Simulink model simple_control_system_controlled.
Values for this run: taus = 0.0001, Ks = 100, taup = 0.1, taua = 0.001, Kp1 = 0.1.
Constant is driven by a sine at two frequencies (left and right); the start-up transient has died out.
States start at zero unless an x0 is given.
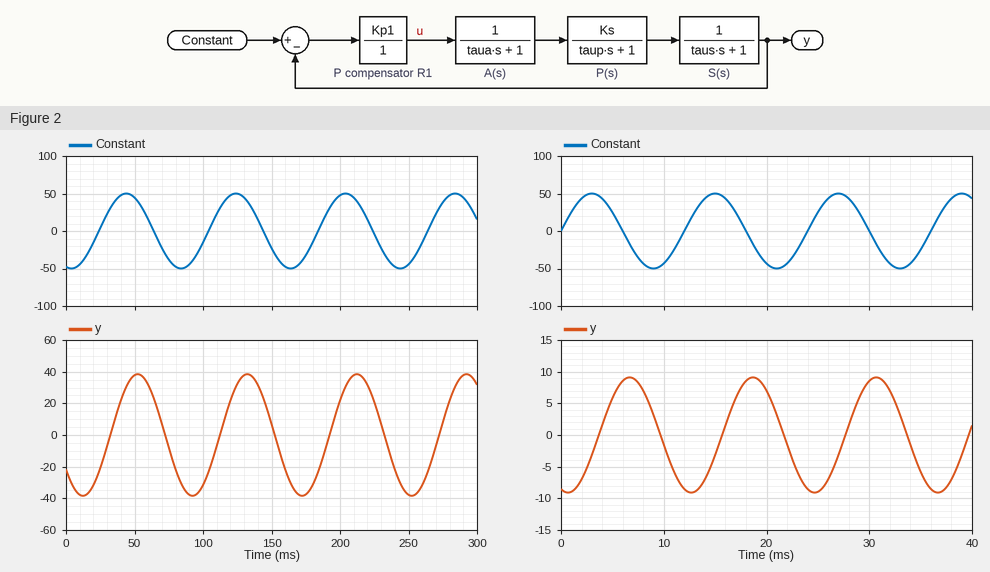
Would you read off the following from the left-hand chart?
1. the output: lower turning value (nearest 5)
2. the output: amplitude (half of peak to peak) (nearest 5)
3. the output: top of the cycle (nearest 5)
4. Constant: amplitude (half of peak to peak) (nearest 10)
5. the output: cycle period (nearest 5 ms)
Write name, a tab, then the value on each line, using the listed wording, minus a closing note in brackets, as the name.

the output: lower turning value	-40
the output: amplitude (half of peak to peak)	40
the output: top of the cycle	40
Constant: amplitude (half of peak to peak)	50
the output: cycle period	80 ms
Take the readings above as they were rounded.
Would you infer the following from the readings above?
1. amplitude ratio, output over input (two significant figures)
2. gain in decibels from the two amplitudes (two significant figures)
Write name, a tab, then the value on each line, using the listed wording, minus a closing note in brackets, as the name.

amplitude ratio, output over input	0.80
gain in decibels from the two amplitudes	-1.9 dB
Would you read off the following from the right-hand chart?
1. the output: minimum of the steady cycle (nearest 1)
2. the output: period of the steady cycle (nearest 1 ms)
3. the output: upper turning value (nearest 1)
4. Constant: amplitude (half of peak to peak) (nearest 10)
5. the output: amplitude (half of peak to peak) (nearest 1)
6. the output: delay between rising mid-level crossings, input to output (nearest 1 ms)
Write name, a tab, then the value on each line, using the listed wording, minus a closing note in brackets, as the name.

the output: minimum of the steady cycle	-9
the output: period of the steady cycle	12 ms
the output: upper turning value	9
Constant: amplitude (half of peak to peak)	50
the output: amplitude (half of peak to peak)	9
the output: delay between rising mid-level crossings, input to output	4 ms
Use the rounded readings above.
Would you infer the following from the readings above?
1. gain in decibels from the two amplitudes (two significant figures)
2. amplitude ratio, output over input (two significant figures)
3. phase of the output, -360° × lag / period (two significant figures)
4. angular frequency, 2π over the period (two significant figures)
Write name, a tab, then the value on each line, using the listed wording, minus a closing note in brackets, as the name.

gain in decibels from the two amplitudes	-15 dB
amplitude ratio, output over input	0.18
phase of the output, -360° × lag / period	-120°
angular frequency, 2π over the period	0.52 rad/ms
